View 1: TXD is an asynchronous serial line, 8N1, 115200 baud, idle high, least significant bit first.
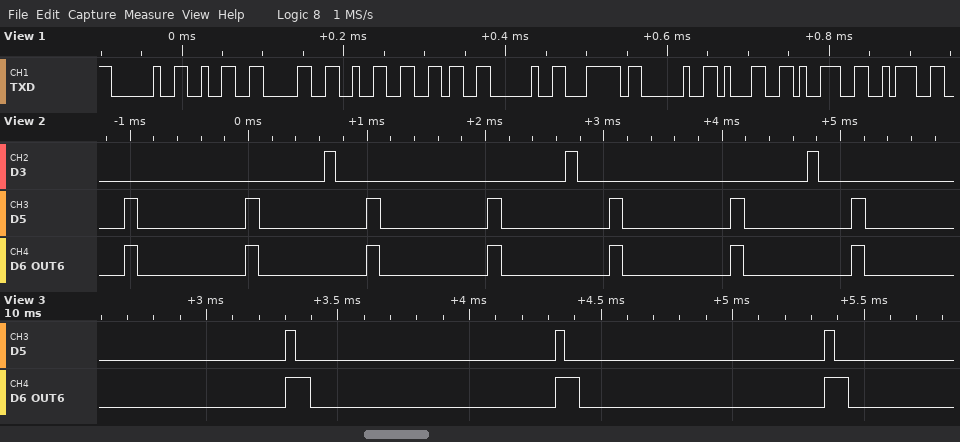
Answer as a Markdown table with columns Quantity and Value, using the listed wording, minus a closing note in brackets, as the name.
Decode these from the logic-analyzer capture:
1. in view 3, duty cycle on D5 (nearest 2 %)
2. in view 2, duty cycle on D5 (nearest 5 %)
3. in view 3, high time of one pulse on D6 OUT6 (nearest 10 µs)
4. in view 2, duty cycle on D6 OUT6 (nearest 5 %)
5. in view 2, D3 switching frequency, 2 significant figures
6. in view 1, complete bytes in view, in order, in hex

| Quantity | Value |
|---|---|
| in view 3, duty cycle on D5 | 4 % |
| in view 2, duty cycle on D5 | 10 % |
| in view 3, high time of one pulse on D6 OUT6 | 90 µs |
| in view 2, duty cycle on D6 OUT6 | 10 % |
| in view 2, D3 switching frequency, 2 significant figures | 490 Hz |
| in view 1, complete bytes in view, in order, in hex | 20 32 30 32 36 20 7C 20 31 39 3A |
